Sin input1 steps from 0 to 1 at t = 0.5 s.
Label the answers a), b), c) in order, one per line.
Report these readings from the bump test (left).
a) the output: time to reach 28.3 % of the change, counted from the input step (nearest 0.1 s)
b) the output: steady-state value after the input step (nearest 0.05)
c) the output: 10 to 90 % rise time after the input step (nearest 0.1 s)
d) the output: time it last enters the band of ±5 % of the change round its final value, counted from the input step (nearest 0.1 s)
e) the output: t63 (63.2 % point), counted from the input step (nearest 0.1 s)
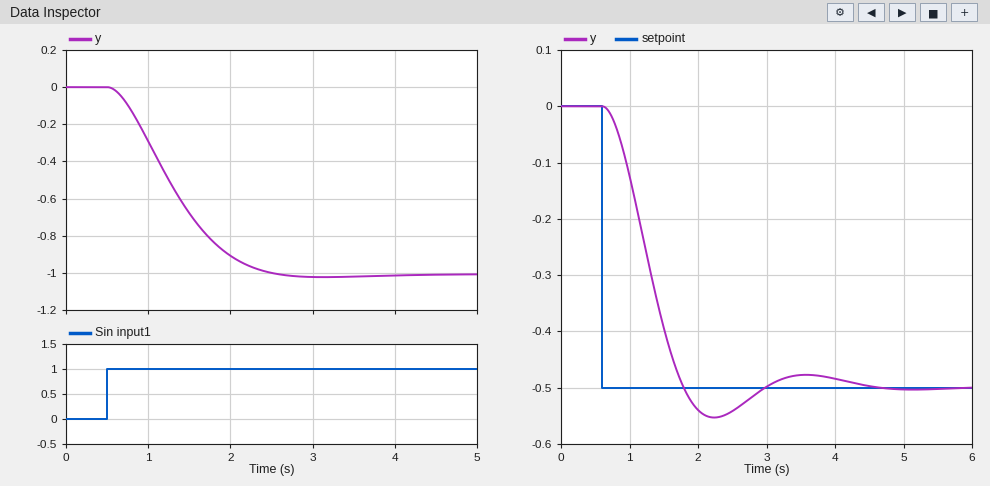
a) 0.5 s
b) -1.00
c) 1.2 s
d) 1.7 s
e) 0.9 s
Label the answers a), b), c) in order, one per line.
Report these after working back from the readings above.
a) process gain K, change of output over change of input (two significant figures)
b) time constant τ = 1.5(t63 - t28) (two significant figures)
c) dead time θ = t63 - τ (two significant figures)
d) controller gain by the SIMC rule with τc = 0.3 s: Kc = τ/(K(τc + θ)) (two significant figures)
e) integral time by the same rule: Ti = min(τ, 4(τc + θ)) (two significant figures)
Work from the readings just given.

a) -1.0
b) 0.60 s
c) 0.30 s
d) -1.0
e) 0.60 s
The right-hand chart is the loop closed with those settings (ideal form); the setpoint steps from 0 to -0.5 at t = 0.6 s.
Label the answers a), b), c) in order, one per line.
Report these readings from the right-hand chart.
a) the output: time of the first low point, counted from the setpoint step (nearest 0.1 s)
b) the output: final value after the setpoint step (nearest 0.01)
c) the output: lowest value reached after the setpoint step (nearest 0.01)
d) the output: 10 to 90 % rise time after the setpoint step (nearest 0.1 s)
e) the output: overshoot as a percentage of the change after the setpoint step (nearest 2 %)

a) 1.6 s
b) -0.50
c) -0.55
d) 0.8 s
e) 10 %
